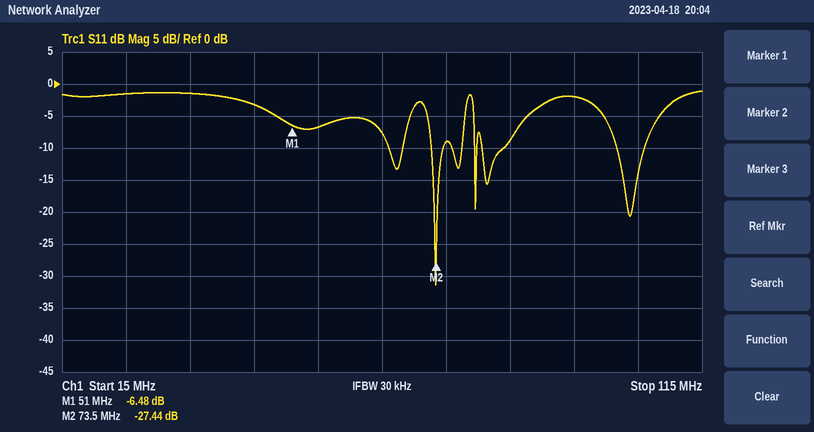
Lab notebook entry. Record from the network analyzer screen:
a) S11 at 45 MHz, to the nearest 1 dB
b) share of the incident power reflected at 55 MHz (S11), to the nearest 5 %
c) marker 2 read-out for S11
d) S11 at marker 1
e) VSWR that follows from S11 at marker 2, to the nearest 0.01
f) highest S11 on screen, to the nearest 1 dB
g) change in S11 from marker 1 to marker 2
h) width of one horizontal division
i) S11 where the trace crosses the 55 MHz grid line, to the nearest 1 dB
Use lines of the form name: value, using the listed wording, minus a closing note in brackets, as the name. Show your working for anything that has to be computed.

S11 at 45 MHz, to the nearest 1 dB: -3 dB
share of the incident power reflected at 55 MHz (S11), to the nearest 5 %: 10^(-7/10) ≈ 20 %
marker 2 read-out for S11: -27.44 dB
S11 at marker 1: -6.48 dB
VSWR that follows from S11 at marker 2, to the nearest 0.01: (1 + 0.0425)/(1 − 0.0425) ≈ 1.09
highest S11 on screen, to the nearest 1 dB: -1 dB
change in S11 from marker 1 to marker 2: -27.44 − (-6.48) = -20.96 dB
width of one horizontal division: 10 MHz
S11 where the trace crosses the 55 MHz grid line, to the nearest 1 dB: -7 dB
